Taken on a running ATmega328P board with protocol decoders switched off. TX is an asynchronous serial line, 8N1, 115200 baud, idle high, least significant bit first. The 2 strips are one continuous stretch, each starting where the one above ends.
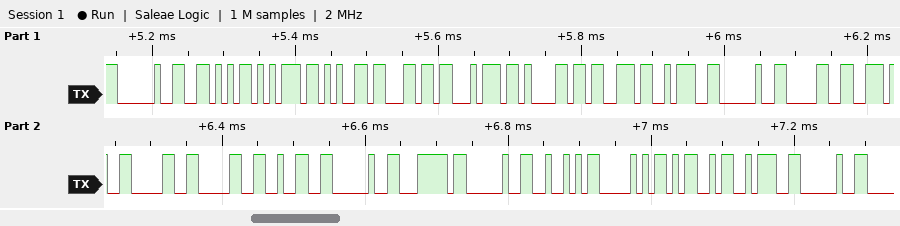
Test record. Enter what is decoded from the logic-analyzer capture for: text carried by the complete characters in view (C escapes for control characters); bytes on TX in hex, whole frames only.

" Vueltas: 0.002 | RPM: "
0x20 0x56 0x75 0x65 0x6C 0x74 0x61 0x73 0x3A 0x20 0x30 0x2E 0x30 0x30 0x32 0x20 0x7C 0x20 0x52 0x50 0x4D 0x3A 0x20
